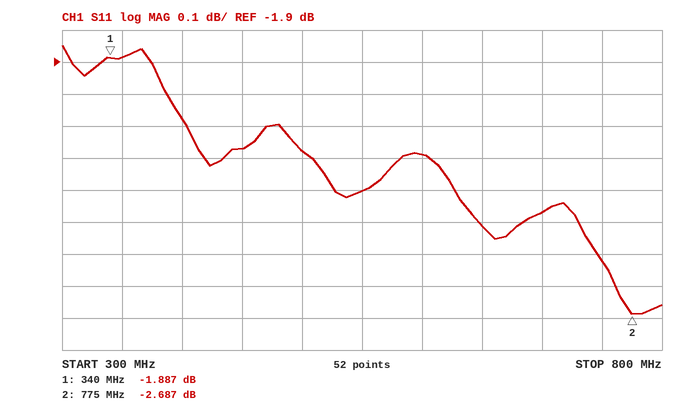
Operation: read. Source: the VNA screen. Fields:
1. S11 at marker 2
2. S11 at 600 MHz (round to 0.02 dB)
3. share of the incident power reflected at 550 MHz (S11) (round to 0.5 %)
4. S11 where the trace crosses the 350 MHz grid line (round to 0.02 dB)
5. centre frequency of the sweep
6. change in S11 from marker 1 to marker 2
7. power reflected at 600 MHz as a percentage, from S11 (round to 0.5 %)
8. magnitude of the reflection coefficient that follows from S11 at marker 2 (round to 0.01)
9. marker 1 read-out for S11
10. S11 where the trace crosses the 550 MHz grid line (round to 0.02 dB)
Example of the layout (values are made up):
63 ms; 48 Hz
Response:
-2.687 dB; -2.18 dB; 59.0 %; -1.88 dB; 550 MHz; -0.800 dB; 60.5 %; 0.73; -1.887 dB; -2.30 dB
